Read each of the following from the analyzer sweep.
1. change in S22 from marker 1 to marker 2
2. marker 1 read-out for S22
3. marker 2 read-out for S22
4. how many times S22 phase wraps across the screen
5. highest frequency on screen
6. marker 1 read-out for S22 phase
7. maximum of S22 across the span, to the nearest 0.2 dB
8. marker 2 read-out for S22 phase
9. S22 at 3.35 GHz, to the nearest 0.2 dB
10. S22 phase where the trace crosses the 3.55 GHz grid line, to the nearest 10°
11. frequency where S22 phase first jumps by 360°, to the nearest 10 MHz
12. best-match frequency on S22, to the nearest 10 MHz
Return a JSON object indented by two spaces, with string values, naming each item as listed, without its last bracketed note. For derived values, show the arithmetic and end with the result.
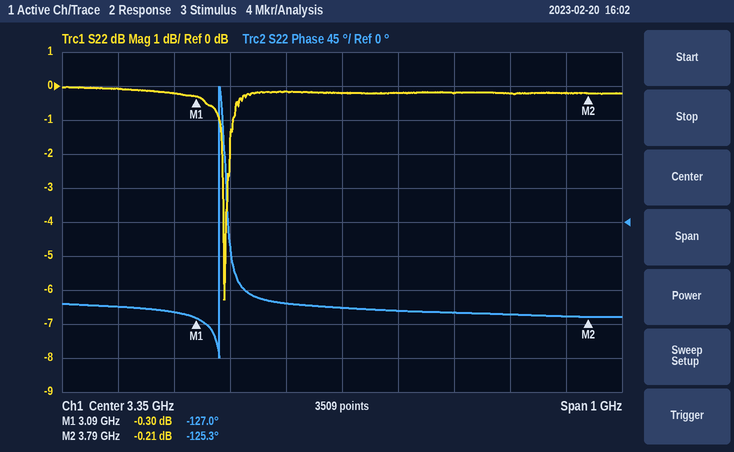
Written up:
{
  "change in S22 from marker 1 to marker 2": "-0.21 − (-0.3) = 0.09 dB",
  "marker 1 read-out for S22": "-0.30 dB",
  "marker 2 read-out for S22": "-0.21 dB",
  "how many times S22 phase wraps across the screen": "1",
  "highest frequency on screen": "3.85 GHz",
  "marker 1 read-out for S22 phase": "-127.0°",
  "maximum of S22 across the span, to the nearest 0.2 dB": "0.0 dB",
  "marker 2 read-out for S22 phase": "-125.3°",
  "S22 at 3.35 GHz, to the nearest 0.2 dB": "-0.2 dB",
  "S22 phase where the trace crosses the 3.55 GHz grid line, to the nearest 10°": "-120°",
  "frequency where S22 phase first jumps by 360°, to the nearest 10 MHz": "3.13 GHz",
  "best-match frequency on S22, to the nearest 10 MHz": "3.14 GHz"
}
